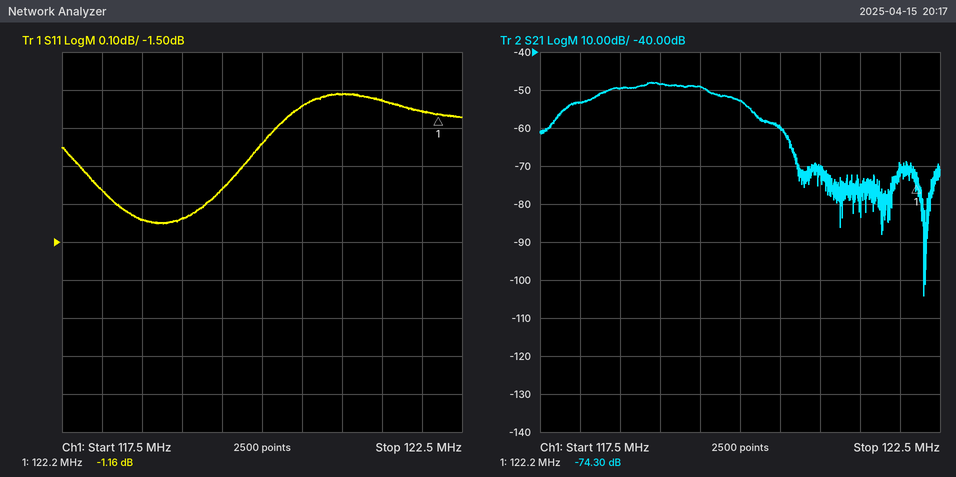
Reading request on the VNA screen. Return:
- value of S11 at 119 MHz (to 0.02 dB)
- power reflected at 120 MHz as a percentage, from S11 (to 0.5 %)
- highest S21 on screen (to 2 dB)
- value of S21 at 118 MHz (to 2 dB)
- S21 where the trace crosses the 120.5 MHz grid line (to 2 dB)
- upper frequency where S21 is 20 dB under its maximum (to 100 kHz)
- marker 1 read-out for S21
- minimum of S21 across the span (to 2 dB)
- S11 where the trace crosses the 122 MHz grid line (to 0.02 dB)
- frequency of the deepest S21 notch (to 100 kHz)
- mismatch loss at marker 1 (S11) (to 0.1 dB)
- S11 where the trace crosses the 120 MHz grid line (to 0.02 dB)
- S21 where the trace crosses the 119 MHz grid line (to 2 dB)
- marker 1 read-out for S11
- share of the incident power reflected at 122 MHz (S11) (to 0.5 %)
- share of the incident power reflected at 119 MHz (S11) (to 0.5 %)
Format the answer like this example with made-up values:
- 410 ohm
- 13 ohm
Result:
- -1.44 dB
- 75.0 %
- -48 dB
- -54 dB
- -60 dB
- 120.7 MHz
- -74.30 dB
- -104 dB
- -1.16 dB
- 122.3 MHz
- 6.3 dB
- -1.24 dB
- -48 dB
- -1.16 dB
- 76.5 %
- 72.0 %
